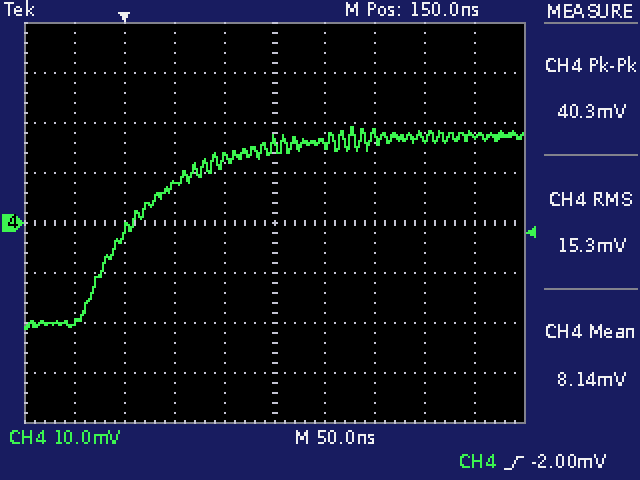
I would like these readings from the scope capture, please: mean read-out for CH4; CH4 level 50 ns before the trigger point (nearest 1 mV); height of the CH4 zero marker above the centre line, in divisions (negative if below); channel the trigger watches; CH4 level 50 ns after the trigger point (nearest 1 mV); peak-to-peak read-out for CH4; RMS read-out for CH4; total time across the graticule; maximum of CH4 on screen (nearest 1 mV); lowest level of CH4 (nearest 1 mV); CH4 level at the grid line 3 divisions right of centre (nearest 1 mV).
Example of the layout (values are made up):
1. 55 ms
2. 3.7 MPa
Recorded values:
1. 8.14 mV
2. -20 mV
3. 0.0 div
4. CH4
5. 8 mV
6. 40.3 mV
7. 15.3 mV
8. 500 ns
9. 19 mV
10. -21 mV
11. 17 mV
